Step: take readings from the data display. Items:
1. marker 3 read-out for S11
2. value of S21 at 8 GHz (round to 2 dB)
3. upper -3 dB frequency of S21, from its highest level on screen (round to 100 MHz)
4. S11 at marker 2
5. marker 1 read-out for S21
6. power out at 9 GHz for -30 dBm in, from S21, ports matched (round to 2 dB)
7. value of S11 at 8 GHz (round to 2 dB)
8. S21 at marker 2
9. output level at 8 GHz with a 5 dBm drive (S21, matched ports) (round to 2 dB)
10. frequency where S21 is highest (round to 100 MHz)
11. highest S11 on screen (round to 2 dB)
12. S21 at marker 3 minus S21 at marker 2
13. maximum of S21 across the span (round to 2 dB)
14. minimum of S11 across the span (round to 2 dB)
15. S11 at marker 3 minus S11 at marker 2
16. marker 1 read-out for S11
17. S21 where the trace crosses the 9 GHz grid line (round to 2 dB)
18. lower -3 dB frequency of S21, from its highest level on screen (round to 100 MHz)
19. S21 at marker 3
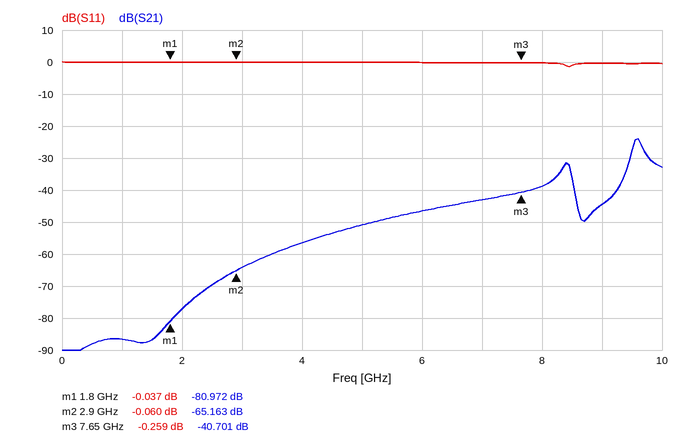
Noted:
-0.259 dB
-38 dB
9.7 GHz
-0.060 dB
-80.972 dB
-74 dBm
0 dB
-65.163 dB
-34 dBm
9.6 GHz
0 dB
24.462 dB
-24 dB
-2 dB
-0.199 dB
-0.037 dB
-44 dB
9.5 GHz
-40.701 dB
